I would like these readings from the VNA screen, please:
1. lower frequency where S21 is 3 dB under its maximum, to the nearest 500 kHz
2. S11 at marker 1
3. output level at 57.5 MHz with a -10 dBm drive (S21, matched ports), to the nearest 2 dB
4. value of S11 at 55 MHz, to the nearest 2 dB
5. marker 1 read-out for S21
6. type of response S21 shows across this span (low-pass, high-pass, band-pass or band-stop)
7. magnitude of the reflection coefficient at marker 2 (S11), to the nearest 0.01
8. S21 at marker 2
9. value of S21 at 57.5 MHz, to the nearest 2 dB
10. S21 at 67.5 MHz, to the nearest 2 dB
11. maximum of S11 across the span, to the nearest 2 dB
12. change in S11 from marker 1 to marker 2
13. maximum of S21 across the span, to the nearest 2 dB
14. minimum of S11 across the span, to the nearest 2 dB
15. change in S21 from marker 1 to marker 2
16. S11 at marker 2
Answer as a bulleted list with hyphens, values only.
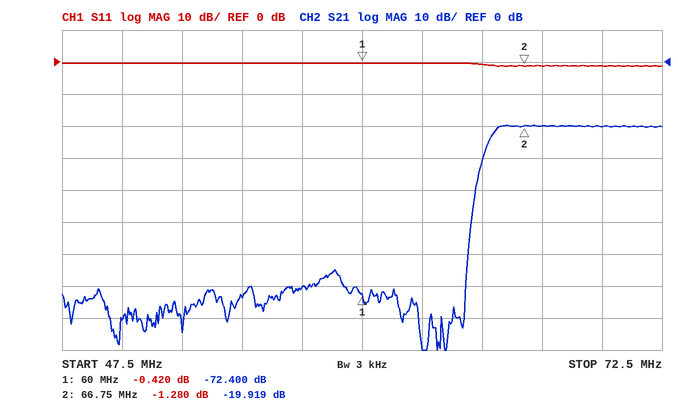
- 65.5 MHz
- -0.420 dB
- -80 dBm
- 0 dB
- -72.400 dB
- high-pass
- 0.86
- -19.919 dB
- -70 dB
- -20 dB
- 0 dB
- -0.860 dB
- -20 dB
- -2 dB
- 52.481 dB
- -1.280 dB
